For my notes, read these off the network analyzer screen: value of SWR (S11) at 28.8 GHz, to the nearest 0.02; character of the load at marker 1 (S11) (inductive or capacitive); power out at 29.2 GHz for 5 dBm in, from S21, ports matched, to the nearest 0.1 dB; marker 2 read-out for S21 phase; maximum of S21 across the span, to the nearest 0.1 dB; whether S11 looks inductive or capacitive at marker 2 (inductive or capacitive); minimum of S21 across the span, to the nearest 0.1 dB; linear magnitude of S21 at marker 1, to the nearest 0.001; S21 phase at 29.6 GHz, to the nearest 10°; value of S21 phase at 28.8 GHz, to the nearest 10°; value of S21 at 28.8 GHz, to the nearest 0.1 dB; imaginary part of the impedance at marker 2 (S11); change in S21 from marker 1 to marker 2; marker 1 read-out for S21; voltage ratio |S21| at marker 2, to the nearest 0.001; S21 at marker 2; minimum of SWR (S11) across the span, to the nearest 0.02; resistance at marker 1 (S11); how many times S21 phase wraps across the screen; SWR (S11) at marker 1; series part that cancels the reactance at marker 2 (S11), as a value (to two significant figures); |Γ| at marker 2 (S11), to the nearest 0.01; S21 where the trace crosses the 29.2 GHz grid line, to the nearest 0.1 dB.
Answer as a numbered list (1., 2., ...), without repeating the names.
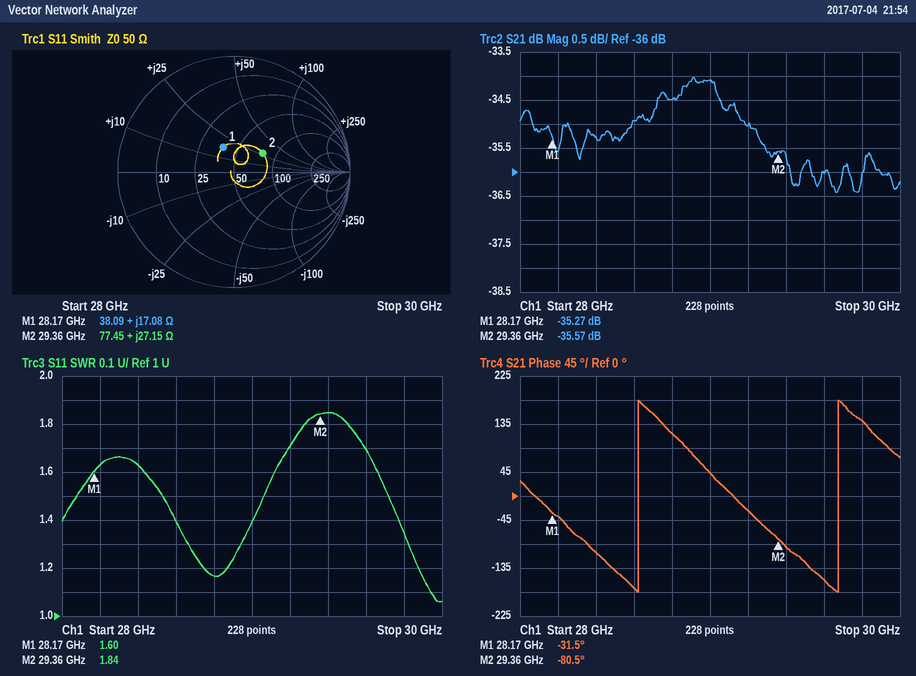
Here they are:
1. 1.16
2. inductive
3. -30.0 dBm
4. -80.5°
5. -34.0 dB
6. inductive
7. -36.4 dB
8. 0.017
9. -160°
10. 120°
11. -34.5 dB
12. +27.15 Ω
13. -0.30 dB
14. -35.27 dB
15. 0.017
16. -35.57 dB
17. 1.06
18. 38.09 Ω
19. 2
20. 1.60
21. 200 fF
22. 0.30
23. -35.0 dB
